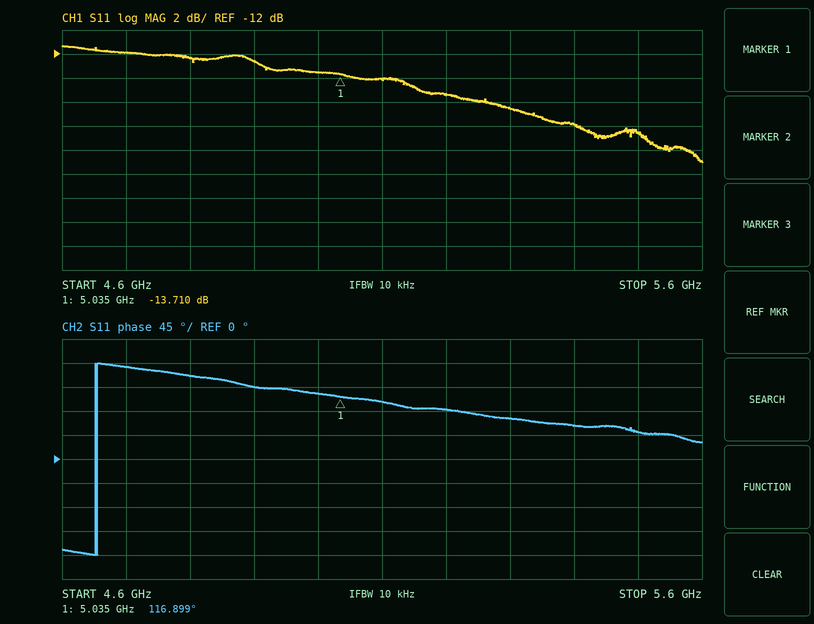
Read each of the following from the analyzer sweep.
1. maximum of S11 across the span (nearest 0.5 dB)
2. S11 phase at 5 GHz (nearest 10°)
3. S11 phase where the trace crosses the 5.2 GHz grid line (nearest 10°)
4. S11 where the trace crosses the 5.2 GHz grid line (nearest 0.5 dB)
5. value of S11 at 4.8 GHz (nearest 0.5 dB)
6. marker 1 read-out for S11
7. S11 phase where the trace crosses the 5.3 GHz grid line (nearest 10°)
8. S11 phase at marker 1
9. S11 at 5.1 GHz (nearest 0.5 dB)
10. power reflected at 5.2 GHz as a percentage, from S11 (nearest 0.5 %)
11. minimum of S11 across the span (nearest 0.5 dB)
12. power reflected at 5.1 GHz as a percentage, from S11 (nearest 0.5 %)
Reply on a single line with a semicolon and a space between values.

-11.5 dB; 120°; 90°; -15.5 dB; -12.5 dB; -13.710 dB; 80°; 116.899°; -14.0 dB; 3.0 %; -21.0 dB; 4.0 %
